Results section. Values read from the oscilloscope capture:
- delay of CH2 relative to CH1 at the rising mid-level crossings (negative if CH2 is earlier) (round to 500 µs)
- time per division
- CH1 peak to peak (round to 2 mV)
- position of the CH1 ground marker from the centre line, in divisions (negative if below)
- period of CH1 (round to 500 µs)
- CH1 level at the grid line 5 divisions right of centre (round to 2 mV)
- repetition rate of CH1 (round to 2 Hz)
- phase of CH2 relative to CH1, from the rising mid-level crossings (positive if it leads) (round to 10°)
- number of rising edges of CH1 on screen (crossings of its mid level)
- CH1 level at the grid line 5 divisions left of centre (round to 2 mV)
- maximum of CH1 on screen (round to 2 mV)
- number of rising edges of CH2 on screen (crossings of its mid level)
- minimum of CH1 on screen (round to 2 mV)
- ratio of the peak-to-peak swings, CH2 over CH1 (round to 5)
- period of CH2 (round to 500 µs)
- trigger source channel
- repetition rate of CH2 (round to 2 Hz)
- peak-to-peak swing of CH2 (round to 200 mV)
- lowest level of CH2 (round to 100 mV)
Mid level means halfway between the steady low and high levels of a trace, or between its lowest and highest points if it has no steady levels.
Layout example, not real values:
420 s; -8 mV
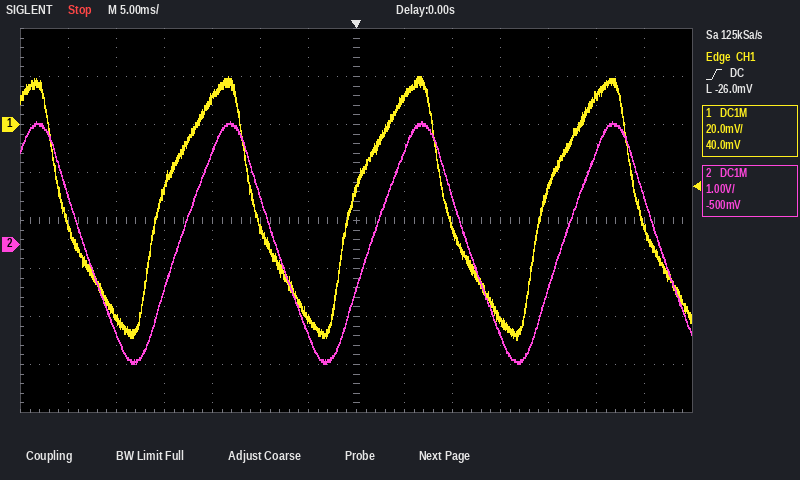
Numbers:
+2.0 ms; 5 ms; 110 mV; +2.0 div; 20.0 ms; 12 mV; 50 Hz; -40°; 3; -82 mV; 20 mV; 3; -90 mV; 45; 20.0 ms; CH1; 50 Hz; 5.0 V; -2.5 V
